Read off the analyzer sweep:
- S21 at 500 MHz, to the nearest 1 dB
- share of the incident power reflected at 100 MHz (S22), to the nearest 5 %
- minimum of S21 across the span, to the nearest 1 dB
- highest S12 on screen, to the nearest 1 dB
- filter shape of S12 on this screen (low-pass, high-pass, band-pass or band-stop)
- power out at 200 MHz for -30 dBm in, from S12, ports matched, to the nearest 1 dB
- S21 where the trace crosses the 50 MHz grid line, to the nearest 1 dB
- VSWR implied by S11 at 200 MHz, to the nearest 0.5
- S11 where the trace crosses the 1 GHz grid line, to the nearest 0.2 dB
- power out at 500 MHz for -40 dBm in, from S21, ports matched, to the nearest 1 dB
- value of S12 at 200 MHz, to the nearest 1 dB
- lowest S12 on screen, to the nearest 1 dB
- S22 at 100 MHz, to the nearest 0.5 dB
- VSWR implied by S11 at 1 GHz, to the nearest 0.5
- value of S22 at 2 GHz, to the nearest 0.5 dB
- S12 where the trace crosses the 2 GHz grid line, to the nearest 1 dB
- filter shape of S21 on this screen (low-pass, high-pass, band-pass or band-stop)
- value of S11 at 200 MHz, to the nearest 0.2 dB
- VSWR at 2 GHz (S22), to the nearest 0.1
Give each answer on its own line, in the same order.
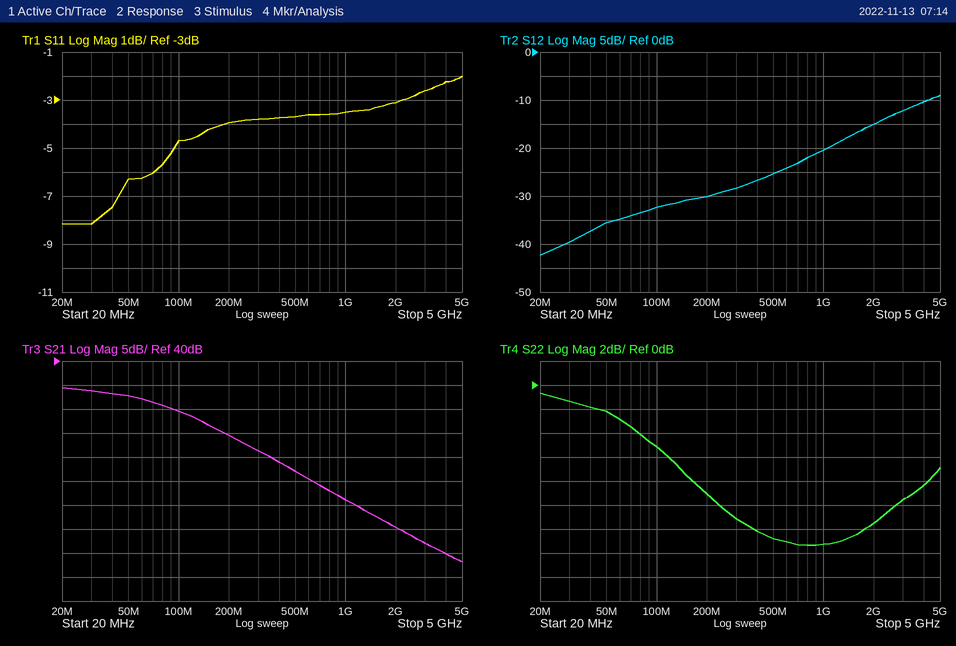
17 dB
30 %
-2 dB
-9 dB
high-pass
-60 dBm
33 dB
4.5
-3.6 dB
-23 dBm
-30 dB
-42 dB
-5.0 dB
5.0
-11.5 dB
-15 dB
low-pass
-4.0 dB
1.7
